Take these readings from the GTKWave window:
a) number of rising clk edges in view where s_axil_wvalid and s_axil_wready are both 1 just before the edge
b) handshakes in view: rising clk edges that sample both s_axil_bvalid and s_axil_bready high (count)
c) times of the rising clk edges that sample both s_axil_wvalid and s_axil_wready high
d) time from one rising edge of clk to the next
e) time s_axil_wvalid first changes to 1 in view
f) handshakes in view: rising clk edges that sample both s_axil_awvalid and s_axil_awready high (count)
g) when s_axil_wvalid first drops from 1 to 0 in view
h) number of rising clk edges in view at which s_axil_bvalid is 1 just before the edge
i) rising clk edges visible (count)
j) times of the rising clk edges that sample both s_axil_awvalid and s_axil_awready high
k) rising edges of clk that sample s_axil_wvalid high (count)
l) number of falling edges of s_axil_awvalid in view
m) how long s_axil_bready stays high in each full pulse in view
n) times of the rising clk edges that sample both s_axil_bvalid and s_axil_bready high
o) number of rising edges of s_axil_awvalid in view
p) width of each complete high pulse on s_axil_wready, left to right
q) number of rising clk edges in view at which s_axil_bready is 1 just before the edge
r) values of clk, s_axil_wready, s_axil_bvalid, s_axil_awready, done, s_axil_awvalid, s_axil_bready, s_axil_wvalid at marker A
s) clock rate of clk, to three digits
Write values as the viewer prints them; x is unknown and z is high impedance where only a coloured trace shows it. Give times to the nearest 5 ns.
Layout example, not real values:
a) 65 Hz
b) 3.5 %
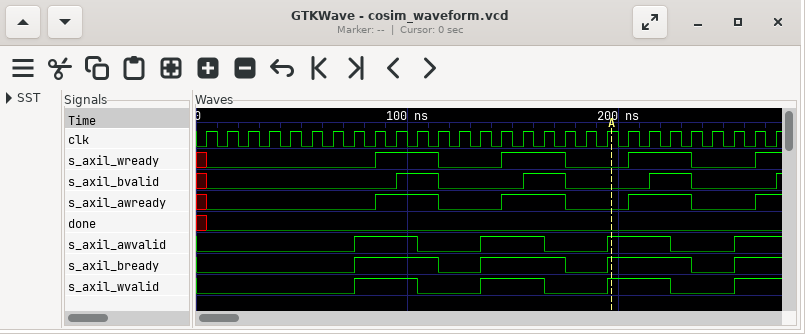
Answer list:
a) 7
b) 6
c) 95 ns, 105 ns, 155 ns, 165 ns, 215 ns, 225 ns, 275 ns
d) 10 ns
e) 75 ns
f) 7
g) 105 ns
h) 6
i) 28
j) 95 ns, 105 ns, 155 ns, 165 ns, 215 ns, 225 ns, 275 ns
k) 11
l) 3
m) 40 ns, 40 ns, 40 ns
n) 105 ns, 115 ns, 165 ns, 175 ns, 225 ns, 235 ns
o) 4
p) 30 ns, 30 ns, 30 ns
q) 14
r) clk=1, s_axil_wready=0, s_axil_bvalid=0, s_axil_awready=0, done=0, s_axil_awvalid=1, s_axil_bready=1, s_axil_wvalid=1
s) 100 MHz
